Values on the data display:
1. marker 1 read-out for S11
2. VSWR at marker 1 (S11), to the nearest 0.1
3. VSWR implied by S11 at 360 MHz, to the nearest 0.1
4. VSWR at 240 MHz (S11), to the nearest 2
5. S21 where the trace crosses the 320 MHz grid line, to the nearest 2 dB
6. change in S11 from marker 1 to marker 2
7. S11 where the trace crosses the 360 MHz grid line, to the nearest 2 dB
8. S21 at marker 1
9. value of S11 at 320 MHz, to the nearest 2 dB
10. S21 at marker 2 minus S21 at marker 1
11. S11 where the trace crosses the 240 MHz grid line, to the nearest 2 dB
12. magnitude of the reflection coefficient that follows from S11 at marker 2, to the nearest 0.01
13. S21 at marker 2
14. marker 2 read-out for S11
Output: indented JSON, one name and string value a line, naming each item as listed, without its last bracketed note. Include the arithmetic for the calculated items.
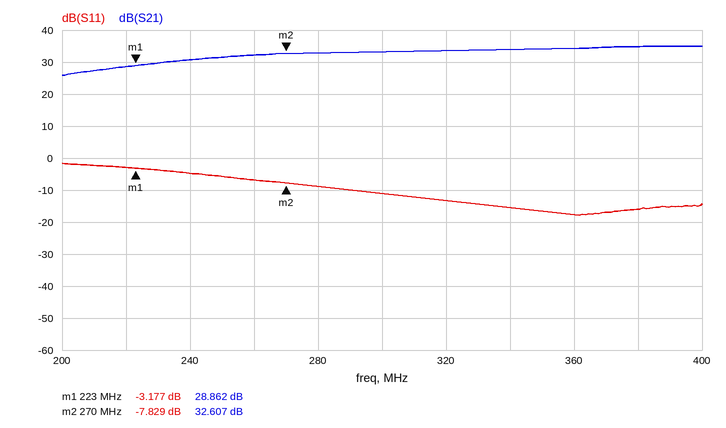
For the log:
{
  "marker 1 read-out for S11": "-3.177 dB",
  "VSWR at marker 1 (S11), to the nearest 0.1": "(1 + 0.6937)/(1 − 0.6937) ≈ 5.5",
  "VSWR implied by S11 at 360 MHz, to the nearest 0.1": "|Γ| = 10^(-18/20) = 0.1259; VSWR = (1 + 0.1259)/(1 − 0.1259) ≈ 1.3",
  "VSWR at 240 MHz (S11), to the nearest 2": "|Γ| = 10^(-4/20) = 0.6310; VSWR = (1 + 0.6310)/(1 − 0.6310) ≈ 4",
  "S21 where the trace crosses the 320 MHz grid line, to the nearest 2 dB": "34 dB",
  "change in S11 from marker 1 to marker 2": "-7.829 − (-3.177) = -4.652 dB",
  "S11 where the trace crosses the 360 MHz grid line, to the nearest 2 dB": "-18 dB",
  "S21 at marker 1": "28.862 dB",
  "value of S11 at 320 MHz, to the nearest 2 dB": "-14 dB",
  "S21 at marker 2 minus S21 at marker 1": "32.607 − (28.862) = 3.745 dB",
  "S11 where the trace crosses the 240 MHz grid line, to the nearest 2 dB": "-4 dB",
  "magnitude of the reflection coefficient that follows from S11 at marker 2, to the nearest 0.01": "10^(-7.829/20) ≈ 0.41",
  "S21 at marker 2": "32.607 dB",
  "marker 2 read-out for S11": "-7.829 dB"
}
